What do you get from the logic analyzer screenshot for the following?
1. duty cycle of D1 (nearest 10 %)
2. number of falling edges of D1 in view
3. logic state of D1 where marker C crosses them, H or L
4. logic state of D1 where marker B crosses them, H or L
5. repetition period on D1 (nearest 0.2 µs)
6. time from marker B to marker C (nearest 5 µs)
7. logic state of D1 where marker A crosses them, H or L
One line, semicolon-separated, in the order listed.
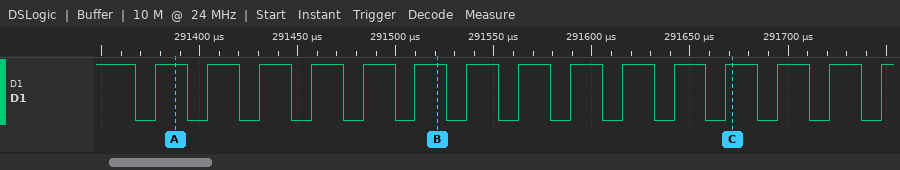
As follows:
60 %; 15; D1=H; D1=H; 26.4 µs; 150 µs; D1=H
